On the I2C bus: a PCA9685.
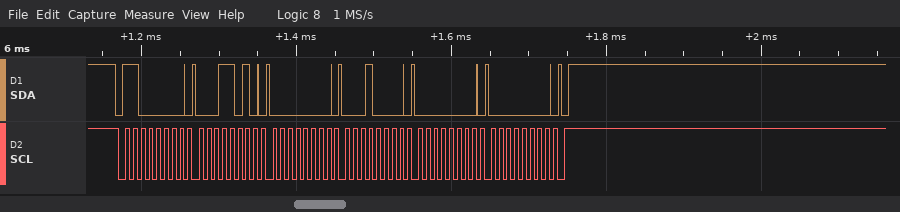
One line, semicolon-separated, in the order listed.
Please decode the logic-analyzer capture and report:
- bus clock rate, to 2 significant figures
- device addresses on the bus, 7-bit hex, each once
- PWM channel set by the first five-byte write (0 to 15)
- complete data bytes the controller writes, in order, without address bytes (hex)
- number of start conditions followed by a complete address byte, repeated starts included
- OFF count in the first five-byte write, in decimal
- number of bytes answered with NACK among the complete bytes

100 kHz; 0x60; 5; 1A 00 10 00 00; 1; 0; 0
